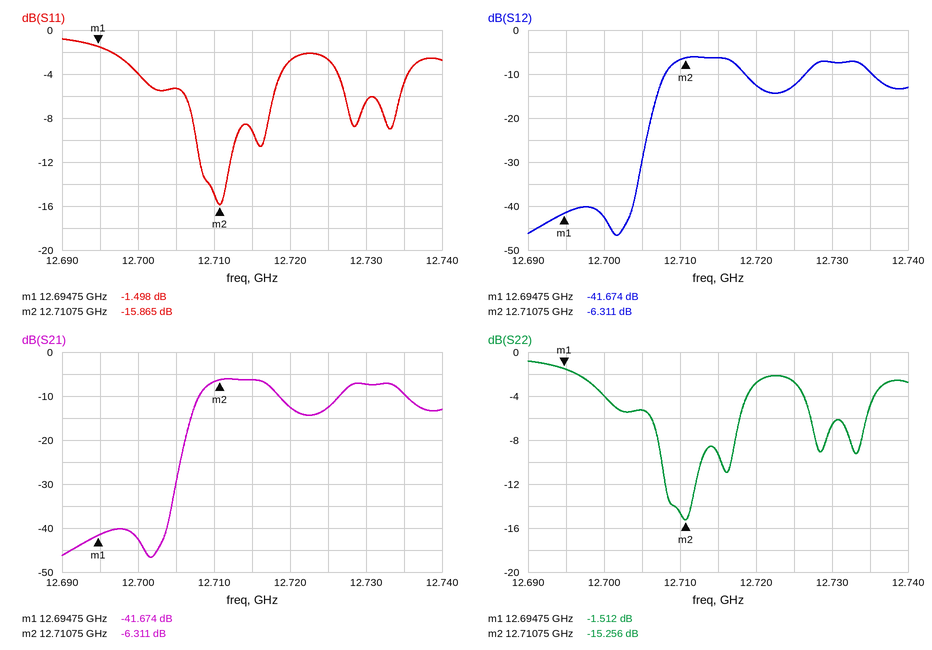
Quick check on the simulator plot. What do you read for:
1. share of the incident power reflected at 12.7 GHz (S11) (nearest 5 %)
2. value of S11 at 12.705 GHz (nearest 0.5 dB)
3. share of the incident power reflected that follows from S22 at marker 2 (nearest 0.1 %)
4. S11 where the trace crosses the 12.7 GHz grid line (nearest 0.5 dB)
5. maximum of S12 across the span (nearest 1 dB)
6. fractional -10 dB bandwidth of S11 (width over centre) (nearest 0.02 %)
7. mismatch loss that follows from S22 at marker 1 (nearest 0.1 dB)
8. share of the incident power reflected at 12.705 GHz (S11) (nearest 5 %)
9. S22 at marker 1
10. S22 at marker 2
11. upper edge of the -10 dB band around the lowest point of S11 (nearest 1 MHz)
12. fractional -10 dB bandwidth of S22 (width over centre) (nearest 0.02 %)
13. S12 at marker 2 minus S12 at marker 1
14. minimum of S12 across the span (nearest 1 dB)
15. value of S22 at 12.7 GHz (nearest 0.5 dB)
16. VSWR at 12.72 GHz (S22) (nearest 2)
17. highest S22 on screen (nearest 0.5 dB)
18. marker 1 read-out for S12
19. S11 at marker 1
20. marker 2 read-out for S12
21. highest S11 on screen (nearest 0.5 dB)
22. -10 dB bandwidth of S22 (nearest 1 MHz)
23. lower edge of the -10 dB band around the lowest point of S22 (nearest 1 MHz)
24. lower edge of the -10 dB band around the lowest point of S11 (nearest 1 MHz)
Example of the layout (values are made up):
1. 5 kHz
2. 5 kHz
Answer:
1. 40 %
2. -5.5 dB
3. 3.0 %
4. -4.0 dB
5. -6 dB
6. 0.04 %
7. 5.3 dB
8. 30 %
9. -1.512 dB
10. -15.256 dB
11. 12.713 GHz
12. 0.04 %
13. 35.363 dB
14. -47 dB
15. -4.0 dB
16. 6
17. -1.0 dB
18. -41.674 dB
19. -1.498 dB
20. -6.311 dB
21. -1.0 dB
22. 5 MHz
23. 12.708 GHz
24. 12.708 GHz
